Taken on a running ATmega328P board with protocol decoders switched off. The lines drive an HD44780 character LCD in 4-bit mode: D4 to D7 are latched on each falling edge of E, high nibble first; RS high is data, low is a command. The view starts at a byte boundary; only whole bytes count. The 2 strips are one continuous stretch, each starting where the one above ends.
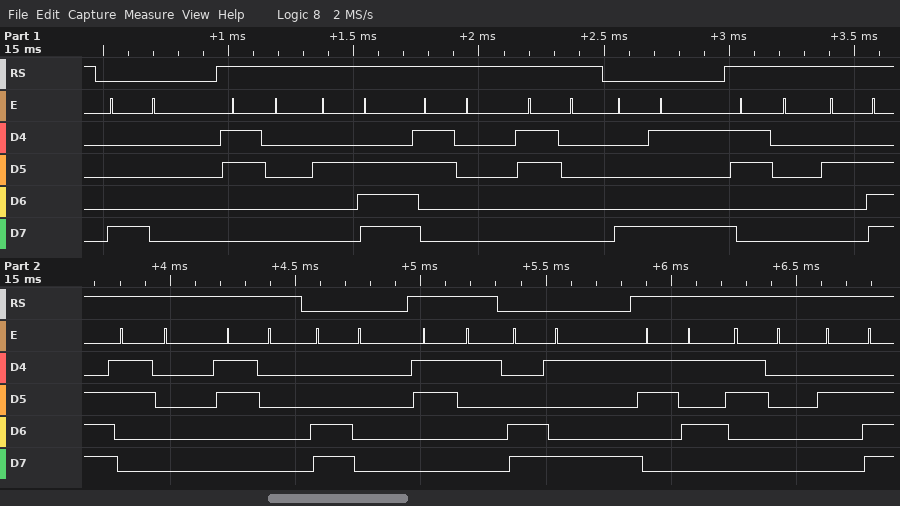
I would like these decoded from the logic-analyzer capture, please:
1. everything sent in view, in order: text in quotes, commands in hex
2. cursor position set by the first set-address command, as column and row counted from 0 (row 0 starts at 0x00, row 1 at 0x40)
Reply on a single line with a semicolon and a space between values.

0x80 "0.00" 0x89 "0.00" 0xC0 "1" 0xC9 "50."; column 0, row 0
